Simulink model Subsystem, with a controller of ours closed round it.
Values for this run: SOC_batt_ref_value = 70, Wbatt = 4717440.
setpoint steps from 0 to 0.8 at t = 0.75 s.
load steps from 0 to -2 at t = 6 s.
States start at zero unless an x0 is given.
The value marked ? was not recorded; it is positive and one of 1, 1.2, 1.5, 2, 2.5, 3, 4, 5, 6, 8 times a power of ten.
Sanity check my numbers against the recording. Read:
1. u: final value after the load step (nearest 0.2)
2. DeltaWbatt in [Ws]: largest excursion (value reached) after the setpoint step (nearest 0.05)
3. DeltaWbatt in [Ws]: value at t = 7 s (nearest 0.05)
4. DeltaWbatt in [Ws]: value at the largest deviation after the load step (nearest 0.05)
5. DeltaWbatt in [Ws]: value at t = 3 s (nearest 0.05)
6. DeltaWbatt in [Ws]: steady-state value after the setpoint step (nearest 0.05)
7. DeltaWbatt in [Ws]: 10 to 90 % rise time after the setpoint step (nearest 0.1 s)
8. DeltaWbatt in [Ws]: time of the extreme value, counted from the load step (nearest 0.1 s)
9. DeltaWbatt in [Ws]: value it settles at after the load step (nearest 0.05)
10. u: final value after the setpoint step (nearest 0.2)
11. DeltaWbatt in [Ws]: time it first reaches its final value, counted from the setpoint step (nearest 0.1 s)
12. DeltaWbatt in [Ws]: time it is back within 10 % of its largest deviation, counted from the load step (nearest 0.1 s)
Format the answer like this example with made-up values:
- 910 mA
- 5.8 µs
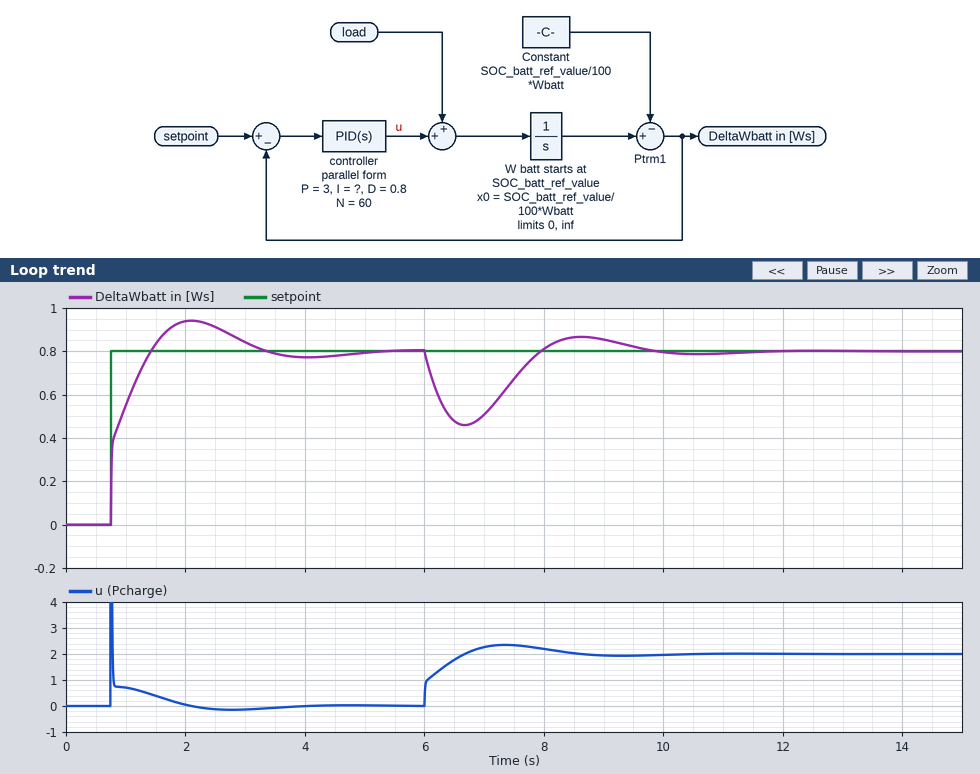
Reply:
- 2.0
- 0.95
- 0.50
- 0.45
- 0.85
- 0.80
- 0.5 s
- 0.7 s
- 0.80
- 0.0
- 0.7 s
- 3.3 s
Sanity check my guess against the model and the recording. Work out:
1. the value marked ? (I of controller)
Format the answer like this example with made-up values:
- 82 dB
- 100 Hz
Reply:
- 6
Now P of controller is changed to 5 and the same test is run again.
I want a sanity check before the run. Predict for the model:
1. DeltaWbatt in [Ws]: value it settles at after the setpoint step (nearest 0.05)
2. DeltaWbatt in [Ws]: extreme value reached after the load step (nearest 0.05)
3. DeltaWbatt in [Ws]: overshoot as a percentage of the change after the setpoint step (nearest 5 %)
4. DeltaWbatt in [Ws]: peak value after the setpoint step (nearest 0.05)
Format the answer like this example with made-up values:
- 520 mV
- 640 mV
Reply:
- 0.80
- 0.55
- 10 %
- 0.90
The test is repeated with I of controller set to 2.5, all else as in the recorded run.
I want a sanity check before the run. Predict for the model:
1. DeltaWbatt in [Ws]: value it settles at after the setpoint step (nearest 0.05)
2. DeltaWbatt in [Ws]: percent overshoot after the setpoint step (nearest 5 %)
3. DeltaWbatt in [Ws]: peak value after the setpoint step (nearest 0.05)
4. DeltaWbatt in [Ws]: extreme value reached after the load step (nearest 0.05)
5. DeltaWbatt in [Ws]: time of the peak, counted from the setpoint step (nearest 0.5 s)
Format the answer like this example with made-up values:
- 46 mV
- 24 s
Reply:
- 0.80
- 10 %
- 0.90
- 0.35
- 2.0 s
